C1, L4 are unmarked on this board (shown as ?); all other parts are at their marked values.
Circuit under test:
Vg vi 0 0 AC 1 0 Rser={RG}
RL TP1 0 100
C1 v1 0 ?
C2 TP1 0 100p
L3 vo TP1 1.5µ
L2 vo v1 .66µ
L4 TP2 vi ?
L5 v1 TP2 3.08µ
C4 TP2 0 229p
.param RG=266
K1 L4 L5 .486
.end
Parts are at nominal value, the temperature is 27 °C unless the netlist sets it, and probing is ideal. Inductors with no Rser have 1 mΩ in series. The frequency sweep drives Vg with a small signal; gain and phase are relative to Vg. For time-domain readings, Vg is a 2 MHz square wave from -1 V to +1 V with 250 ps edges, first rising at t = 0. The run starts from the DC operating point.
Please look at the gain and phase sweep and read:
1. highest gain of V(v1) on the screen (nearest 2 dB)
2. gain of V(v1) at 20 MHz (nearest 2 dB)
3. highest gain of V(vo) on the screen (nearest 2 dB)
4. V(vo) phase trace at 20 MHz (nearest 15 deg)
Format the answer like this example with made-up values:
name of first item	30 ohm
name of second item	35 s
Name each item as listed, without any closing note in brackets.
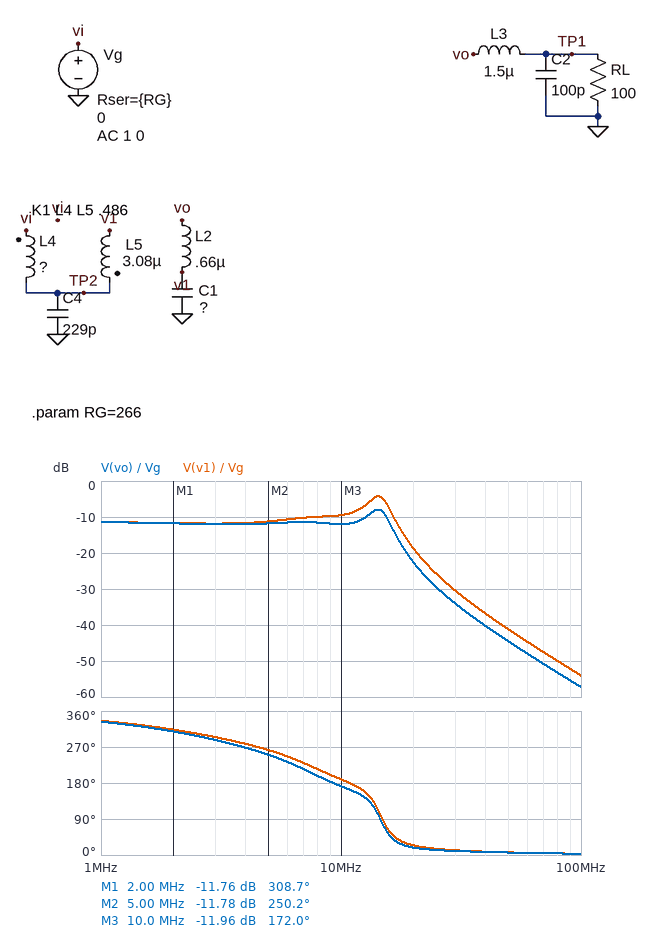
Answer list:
highest gain of V(v1) on the screen	-4 dB
gain of V(v1) at 20 MHz	-18 dB
highest gain of V(vo) on the screen	-8 dB
V(vo) phase trace at 20 MHz	15 deg
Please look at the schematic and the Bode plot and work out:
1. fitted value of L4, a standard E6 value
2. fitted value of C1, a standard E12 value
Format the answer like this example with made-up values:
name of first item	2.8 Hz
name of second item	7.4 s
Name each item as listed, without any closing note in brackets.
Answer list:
fitted value of L4, a standard E6 value	10 µH
fitted value of C1, a standard E12 value	150 pF
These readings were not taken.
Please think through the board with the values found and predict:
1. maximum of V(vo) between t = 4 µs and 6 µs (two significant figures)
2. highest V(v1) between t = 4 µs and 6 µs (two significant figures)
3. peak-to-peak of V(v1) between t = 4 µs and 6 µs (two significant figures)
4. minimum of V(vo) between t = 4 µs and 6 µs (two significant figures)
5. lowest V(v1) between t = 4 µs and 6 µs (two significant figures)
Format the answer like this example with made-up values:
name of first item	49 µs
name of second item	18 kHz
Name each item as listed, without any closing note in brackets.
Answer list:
maximum of V(vo) between t = 4 µs and 6 µs	420 mV
highest V(v1) between t = 4 µs and 6 µs	470 mV
peak-to-peak of V(v1) between t = 4 µs and 6 µs	940 mV
minimum of V(vo) between t = 4 µs and 6 µs	-420 mV
lowest V(v1) between t = 4 µs and 6 µs	-470 mV
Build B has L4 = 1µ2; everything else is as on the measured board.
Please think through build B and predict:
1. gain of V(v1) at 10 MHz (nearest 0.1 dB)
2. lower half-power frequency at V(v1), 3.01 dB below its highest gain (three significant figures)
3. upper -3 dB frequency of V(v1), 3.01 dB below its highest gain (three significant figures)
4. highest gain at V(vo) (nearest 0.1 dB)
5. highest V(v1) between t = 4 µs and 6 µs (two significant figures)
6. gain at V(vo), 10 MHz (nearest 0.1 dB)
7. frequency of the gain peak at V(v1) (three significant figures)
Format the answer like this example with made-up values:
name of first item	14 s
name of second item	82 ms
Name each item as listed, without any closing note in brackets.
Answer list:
gain of V(v1) at 10 MHz	-8.6 dB
lower half-power frequency at V(v1), 3.01 dB below its highest gain	9.86 MHz
upper -3 dB frequency of V(v1), 3.01 dB below its highest gain	15.3 MHz
highest gain at V(vo)	-9.2 dB
highest V(v1) between t = 4 µs and 6 µs	410 mV
gain at V(vo), 10 MHz	-11.1 dB
frequency of the gain peak at V(v1)	13.1 MHz
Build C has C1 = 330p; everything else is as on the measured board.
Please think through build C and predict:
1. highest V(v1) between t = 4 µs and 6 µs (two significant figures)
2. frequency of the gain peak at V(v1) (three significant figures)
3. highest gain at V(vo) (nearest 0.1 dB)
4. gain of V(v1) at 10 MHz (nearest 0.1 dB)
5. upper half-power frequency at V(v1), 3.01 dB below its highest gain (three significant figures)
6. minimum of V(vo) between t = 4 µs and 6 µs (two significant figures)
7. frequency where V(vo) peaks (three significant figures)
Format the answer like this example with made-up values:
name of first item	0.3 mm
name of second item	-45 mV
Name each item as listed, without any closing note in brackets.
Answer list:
highest V(v1) between t = 4 µs and 6 µs	390 mV
frequency of the gain peak at V(v1)	10.9 MHz
highest gain at V(vo)	-10.3 dB
gain of V(v1) at 10 MHz	-8.3 dB
upper half-power frequency at V(v1), 3.01 dB below its highest gain	12.3 MHz
minimum of V(vo) between t = 4 µs and 6 µs	-370 mV
frequency where V(vo) peaks	10.7 MHz
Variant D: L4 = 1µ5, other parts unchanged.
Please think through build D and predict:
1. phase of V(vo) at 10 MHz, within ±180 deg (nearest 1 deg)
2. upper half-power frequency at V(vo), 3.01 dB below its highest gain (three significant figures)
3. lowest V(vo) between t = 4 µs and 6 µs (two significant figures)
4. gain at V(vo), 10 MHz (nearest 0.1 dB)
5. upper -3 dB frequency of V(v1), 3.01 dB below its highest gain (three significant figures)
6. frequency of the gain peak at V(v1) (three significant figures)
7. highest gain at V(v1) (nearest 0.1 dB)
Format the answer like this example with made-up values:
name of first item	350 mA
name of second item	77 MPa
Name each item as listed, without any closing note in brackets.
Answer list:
phase of V(vo) at 10 MHz, within ±180 deg	-150 deg
upper half-power frequency at V(vo), 3.01 dB below its highest gain	15.3 MHz
lowest V(vo) between t = 4 µs and 6 µs	-360 mV
gain at V(vo), 10 MHz	-10.9 dB
upper -3 dB frequency of V(v1), 3.01 dB below its highest gain	15.4 MHz
frequency of the gain peak at V(v1)	13.2 MHz
highest gain at V(v1)	-5.5 dB
